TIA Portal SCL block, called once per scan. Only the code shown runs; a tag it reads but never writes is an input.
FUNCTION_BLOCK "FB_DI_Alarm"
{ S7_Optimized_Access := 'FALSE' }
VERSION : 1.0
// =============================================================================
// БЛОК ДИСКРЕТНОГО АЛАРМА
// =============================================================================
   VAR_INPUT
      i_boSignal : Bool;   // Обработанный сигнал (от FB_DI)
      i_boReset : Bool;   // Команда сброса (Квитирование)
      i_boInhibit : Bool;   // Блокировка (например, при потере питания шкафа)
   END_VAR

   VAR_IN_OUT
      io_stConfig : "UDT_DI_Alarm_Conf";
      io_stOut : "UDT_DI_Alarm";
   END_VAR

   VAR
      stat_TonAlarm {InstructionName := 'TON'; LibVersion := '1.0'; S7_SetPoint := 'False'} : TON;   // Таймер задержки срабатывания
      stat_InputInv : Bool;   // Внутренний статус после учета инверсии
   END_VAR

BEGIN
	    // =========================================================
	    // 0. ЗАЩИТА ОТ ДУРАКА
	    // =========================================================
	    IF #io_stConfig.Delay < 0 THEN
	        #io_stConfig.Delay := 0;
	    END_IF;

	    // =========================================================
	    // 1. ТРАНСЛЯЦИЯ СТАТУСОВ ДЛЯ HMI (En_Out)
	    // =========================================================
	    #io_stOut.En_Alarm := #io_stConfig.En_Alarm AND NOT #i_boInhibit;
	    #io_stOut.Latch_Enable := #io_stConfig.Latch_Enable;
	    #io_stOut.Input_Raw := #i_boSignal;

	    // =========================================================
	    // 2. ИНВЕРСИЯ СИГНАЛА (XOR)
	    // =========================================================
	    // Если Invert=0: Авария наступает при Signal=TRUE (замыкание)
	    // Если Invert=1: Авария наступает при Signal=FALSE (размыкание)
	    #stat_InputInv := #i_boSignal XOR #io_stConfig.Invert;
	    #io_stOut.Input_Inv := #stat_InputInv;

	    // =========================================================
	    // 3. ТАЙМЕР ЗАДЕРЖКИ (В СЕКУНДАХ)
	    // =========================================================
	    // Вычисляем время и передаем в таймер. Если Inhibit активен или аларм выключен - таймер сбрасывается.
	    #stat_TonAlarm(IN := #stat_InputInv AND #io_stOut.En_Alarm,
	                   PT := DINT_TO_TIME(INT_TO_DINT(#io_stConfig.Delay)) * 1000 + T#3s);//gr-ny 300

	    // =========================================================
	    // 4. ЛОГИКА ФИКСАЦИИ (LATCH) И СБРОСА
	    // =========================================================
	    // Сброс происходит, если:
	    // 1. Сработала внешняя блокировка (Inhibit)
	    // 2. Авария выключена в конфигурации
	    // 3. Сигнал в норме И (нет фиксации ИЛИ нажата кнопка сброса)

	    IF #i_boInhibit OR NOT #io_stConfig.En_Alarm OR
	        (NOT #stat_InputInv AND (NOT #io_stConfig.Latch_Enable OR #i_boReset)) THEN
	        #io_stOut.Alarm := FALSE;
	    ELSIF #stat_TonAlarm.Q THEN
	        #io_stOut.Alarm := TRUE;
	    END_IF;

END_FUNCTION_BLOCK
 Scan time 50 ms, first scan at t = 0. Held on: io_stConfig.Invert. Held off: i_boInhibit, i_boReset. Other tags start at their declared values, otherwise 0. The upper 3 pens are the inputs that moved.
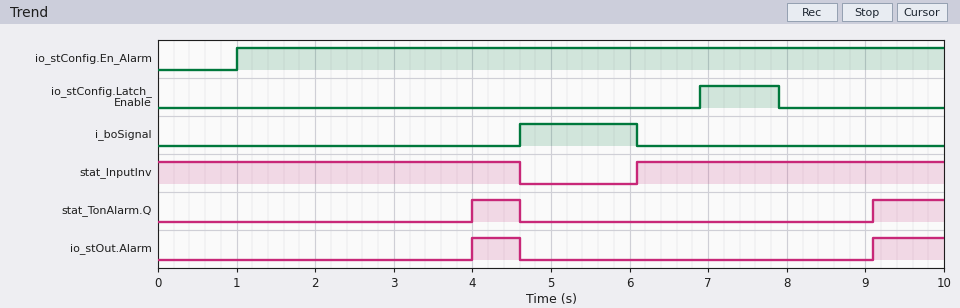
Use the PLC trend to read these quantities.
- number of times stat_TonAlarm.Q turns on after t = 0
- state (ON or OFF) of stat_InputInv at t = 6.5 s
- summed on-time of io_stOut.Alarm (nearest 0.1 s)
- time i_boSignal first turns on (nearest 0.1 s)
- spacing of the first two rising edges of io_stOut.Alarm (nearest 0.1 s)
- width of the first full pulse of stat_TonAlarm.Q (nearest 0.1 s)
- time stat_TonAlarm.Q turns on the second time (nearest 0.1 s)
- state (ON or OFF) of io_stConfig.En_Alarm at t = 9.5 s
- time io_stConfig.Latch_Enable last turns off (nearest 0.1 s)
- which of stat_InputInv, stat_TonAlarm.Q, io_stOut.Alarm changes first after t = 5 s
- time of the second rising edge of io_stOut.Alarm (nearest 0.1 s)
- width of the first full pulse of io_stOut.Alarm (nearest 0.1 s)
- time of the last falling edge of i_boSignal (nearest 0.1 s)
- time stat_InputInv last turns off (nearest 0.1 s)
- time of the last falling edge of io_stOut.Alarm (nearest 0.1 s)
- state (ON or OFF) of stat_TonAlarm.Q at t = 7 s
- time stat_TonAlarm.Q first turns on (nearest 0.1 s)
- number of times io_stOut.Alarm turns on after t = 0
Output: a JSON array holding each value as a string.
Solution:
["2", "ON", "1.5 s", "4.6 s", "5.1 s", "0.6 s", "9.1 s", "ON", "7.9 s", "stat_InputInv", "9.1 s", "0.6 s", "6.1 s", "4.6 s", "4.6 s", "OFF", "4.0 s", "2"]
